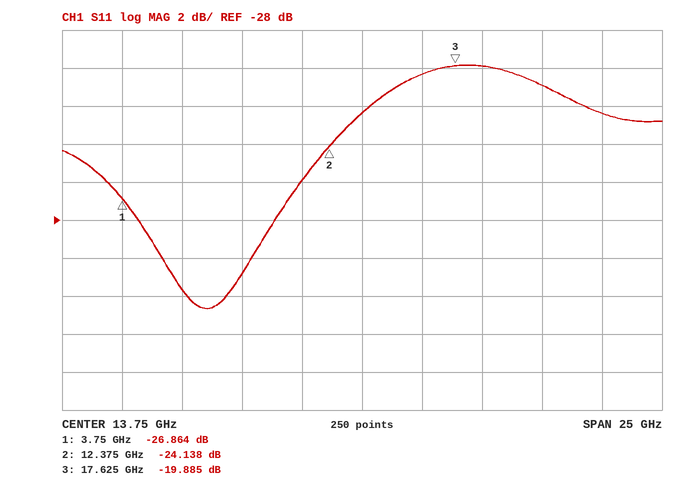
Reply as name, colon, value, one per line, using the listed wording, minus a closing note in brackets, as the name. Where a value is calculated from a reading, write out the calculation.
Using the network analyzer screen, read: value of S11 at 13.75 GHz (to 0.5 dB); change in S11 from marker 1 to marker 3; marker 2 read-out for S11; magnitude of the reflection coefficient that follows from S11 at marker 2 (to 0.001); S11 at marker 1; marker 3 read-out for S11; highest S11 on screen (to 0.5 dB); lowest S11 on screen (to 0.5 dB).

value of S11 at 13.75 GHz: -22.5 dB
change in S11 from marker 1 to marker 3: -19.885 − (-26.864) = 6.979 dB
marker 2 read-out for S11: -24.138 dB
magnitude of the reflection coefficient that follows from S11 at marker 2: 10^(-24.138/20) ≈ 0.062
S11 at marker 1: -26.864 dB
marker 3 read-out for S11: -19.885 dB
highest S11 on screen: -20.0 dB
lowest S11 on screen: -32.5 dB
